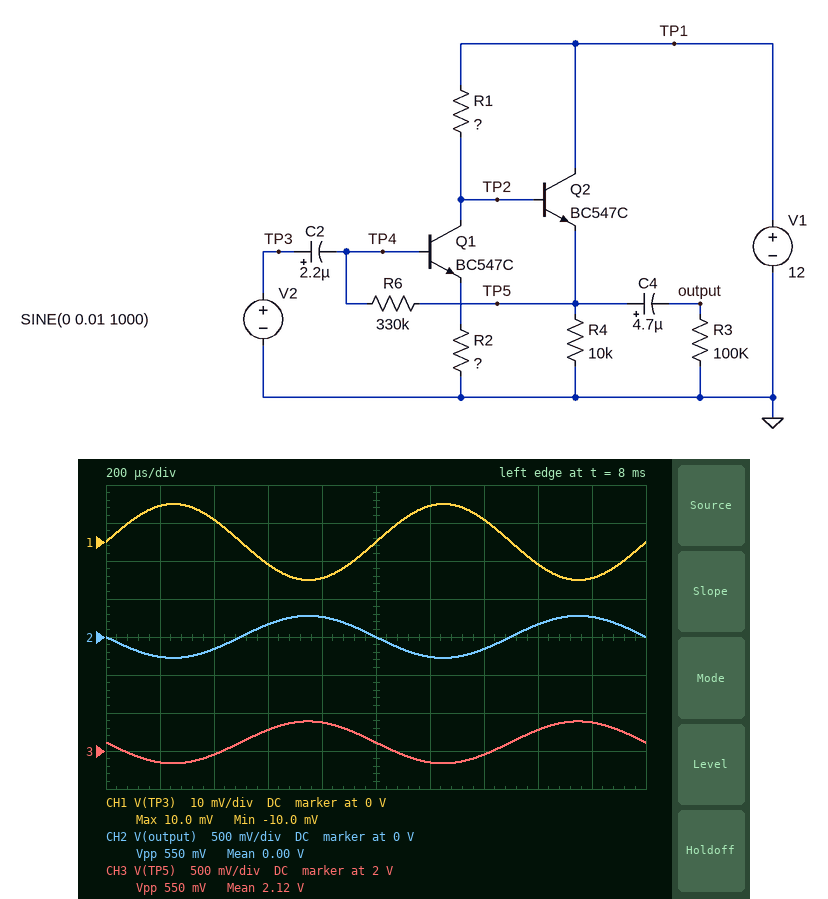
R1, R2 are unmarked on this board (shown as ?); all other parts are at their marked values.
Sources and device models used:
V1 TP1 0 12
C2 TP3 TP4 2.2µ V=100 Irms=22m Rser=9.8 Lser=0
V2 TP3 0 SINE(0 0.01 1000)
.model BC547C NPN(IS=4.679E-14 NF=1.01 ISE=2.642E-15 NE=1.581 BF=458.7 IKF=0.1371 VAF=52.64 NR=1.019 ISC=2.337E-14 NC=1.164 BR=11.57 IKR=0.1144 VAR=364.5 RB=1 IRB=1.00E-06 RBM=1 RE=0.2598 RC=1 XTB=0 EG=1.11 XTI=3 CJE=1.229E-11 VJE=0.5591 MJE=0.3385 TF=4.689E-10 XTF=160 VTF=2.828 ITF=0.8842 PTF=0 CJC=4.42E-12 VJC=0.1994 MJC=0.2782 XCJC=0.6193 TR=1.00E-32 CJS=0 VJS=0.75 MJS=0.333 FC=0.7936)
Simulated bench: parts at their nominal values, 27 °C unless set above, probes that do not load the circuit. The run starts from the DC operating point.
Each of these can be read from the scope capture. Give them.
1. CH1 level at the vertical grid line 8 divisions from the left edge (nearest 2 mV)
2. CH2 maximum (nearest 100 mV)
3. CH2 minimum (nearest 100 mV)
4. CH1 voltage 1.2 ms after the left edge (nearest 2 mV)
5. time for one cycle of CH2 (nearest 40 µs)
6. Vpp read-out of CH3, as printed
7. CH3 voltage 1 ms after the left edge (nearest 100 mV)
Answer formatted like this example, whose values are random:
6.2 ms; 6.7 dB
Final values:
-6 mV; 300 mV; -300 mV; 10 mV; 1.00 ms; 550 mV; 2.1 V
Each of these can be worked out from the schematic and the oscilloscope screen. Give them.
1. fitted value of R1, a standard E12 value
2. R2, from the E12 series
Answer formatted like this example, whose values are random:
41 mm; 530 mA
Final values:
5.6 kΩ; 180 Ω
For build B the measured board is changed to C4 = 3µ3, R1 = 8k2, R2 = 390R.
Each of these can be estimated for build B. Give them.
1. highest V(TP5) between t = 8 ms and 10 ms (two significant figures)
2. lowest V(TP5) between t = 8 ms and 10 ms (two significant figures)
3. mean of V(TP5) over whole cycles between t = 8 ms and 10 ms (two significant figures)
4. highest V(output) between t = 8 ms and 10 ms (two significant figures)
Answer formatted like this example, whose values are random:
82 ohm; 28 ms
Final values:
2.1 V; 1.7 V; 1.9 V; 190 mV
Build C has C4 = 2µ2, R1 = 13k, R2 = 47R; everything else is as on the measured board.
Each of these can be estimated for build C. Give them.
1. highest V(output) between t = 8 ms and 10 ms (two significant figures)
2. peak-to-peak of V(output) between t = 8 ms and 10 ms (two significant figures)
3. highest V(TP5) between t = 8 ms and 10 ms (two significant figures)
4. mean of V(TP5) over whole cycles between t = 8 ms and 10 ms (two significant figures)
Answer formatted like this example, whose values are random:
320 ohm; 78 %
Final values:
1.4 V; 2.5 V; 2.6 V; 1.2 V
